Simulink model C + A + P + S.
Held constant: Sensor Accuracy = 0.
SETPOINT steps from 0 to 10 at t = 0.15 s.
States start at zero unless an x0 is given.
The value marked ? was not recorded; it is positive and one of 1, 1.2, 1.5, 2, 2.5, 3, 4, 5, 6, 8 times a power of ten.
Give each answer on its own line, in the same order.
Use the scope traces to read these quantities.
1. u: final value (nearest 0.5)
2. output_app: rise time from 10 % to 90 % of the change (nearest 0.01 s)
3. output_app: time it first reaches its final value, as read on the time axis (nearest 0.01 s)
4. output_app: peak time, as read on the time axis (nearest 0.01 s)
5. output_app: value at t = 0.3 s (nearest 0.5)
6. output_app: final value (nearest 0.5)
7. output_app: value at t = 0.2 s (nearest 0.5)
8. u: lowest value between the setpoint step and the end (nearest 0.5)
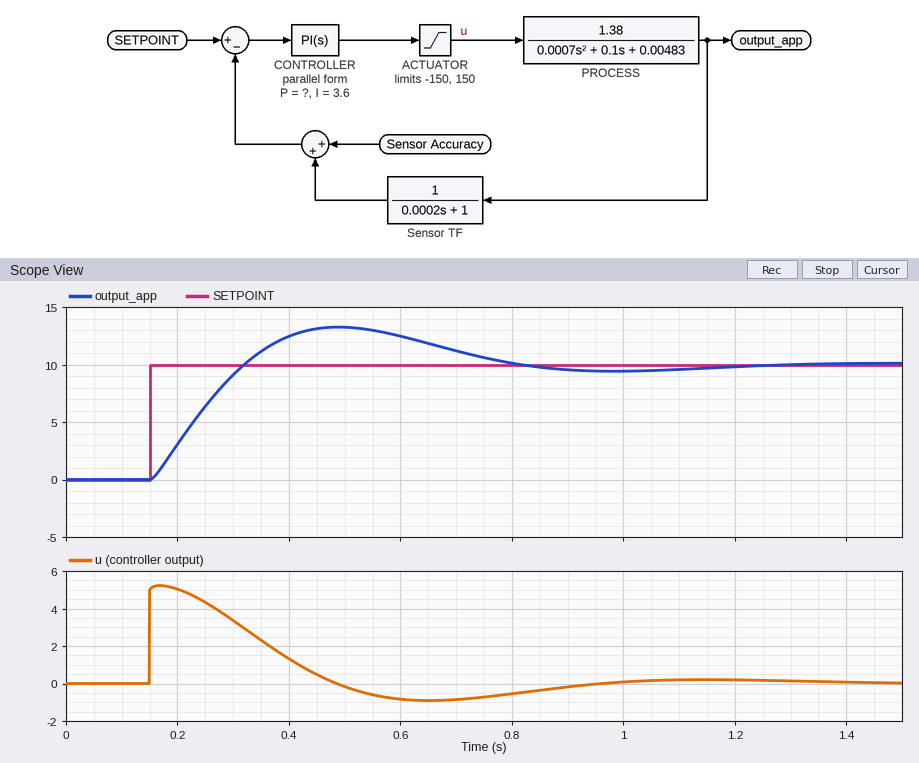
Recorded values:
0.0
0.13 s
0.32 s
0.49 s
9.0
10.0
3.0
-1.0
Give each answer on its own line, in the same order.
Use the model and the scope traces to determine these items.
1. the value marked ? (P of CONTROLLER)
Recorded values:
0.5
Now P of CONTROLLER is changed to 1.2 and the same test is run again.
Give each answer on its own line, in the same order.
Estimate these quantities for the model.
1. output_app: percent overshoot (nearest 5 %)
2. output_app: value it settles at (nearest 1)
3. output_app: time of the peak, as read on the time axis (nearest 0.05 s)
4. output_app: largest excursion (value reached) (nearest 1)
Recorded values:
10 %
10
0.40 s
11
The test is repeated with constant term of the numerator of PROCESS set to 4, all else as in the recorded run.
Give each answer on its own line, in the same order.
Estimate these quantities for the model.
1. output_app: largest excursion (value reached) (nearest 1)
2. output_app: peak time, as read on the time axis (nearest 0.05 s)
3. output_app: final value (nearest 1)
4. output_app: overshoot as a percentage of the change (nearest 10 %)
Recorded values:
12
0.30 s
10
20 %
